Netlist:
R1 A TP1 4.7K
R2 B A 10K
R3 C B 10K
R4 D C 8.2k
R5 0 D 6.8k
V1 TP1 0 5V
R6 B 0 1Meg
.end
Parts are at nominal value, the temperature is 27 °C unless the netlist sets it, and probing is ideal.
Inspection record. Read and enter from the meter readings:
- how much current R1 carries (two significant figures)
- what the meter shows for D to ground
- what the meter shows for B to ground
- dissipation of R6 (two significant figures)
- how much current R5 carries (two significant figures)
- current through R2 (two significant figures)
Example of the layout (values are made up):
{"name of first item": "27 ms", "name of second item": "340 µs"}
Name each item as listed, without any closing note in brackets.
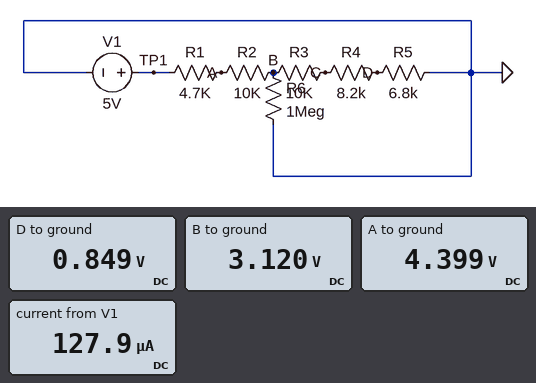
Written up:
{"how much current R1 carries": "130 µA", "what the meter shows for D to ground": "0.849 V", "what the meter shows for B to ground": "3.120 V", "dissipation of R6": "9.7 µW", "how much current R5 carries": "120 µA", "current through R2": "130 µA"}
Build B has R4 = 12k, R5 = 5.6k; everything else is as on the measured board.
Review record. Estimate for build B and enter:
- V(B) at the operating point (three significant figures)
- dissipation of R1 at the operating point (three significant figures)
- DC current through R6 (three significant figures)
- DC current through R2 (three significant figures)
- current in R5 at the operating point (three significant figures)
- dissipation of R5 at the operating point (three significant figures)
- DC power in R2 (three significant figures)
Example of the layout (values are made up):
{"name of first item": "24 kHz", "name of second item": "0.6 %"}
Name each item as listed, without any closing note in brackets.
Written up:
{"V(B) at the operating point": "3.23 V", "dissipation of R1 at the operating point": "68.0 µW", "DC current through R6": "3.23 µA", "DC current through R2": "120 µA", "current in R5 at the operating point": "117 µA", "dissipation of R5 at the operating point": "76.8 µW", "DC power in R2": "145 µW"}
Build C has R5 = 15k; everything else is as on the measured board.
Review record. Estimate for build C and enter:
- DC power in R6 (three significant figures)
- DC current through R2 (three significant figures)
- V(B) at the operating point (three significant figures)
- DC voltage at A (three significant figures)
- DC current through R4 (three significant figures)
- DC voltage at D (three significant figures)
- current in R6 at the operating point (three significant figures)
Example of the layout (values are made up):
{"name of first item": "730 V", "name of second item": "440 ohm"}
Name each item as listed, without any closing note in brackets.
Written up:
{"DC power in R6": "11.8 µW", "DC current through R2": "107 µA", "V(B) at the operating point": "3.43 V", "DC voltage at A": "4.50 V", "DC current through R4": "103 µA", "DC voltage at D": "1.55 V", "current in R6 at the operating point": "3.43 µA"}
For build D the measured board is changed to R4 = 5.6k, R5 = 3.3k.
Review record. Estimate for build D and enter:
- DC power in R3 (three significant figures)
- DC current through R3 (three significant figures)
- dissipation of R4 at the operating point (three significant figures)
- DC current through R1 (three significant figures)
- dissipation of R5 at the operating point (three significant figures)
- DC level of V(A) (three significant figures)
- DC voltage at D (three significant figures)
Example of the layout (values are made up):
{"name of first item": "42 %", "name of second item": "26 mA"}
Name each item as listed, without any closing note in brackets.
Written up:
{"DC power in R3": "218 µW", "DC current through R3": "148 µA", "dissipation of R4 at the operating point": "122 µW", "DC current through R1": "150 µA", "dissipation of R5 at the operating point": "71.9 µW", "DC level of V(A)": "4.29 V", "DC voltage at D": "487 mV"}
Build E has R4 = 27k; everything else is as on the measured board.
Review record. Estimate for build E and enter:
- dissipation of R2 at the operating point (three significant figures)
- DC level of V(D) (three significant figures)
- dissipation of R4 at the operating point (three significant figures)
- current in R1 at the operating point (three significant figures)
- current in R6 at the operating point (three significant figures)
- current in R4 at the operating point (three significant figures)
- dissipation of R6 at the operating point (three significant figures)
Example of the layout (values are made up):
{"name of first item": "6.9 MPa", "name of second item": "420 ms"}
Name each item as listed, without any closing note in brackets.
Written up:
{"dissipation of R2 at the operating point": "77.9 µW", "DC level of V(D)": "575 mV", "dissipation of R4 at the operating point": "193 µW", "current in R1 at the operating point": "88.2 µA", "current in R6 at the operating point": "3.70 µA", "current in R4 at the operating point": "84.5 µA", "dissipation of R6 at the operating point": "13.7 µW"}
